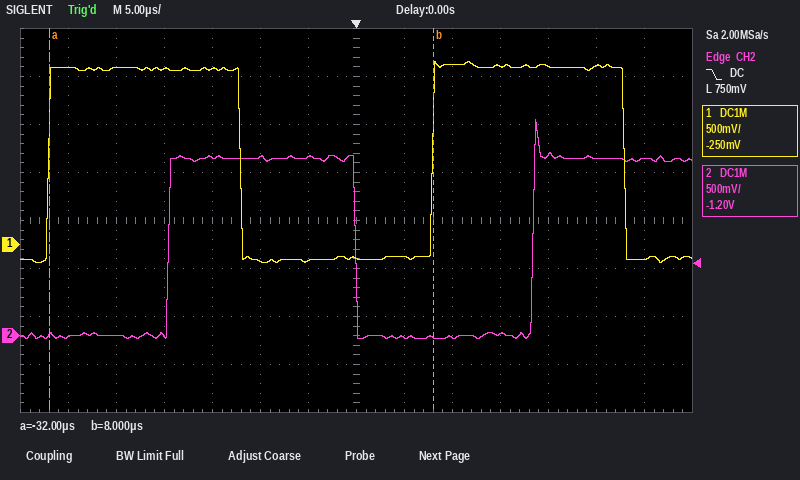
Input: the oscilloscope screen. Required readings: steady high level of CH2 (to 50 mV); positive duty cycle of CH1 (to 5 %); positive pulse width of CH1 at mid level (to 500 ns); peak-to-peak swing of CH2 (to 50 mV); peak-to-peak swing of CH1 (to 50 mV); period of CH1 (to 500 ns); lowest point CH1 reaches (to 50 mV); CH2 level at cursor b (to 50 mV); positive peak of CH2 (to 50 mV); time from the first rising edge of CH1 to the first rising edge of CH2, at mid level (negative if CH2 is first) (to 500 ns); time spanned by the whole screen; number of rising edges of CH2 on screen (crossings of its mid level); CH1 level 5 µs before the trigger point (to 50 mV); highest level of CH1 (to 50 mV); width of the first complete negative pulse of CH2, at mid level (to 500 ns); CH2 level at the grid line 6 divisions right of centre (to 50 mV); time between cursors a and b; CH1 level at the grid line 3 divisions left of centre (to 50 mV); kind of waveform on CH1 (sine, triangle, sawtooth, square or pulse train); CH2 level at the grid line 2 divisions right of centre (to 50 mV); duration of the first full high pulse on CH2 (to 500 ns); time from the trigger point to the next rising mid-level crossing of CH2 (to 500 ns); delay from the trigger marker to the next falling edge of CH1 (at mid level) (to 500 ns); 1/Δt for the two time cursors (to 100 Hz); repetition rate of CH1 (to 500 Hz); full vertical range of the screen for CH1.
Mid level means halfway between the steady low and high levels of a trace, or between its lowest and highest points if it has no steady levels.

1.85 V
50 %
20.0 µs
2.30 V
2.10 V
40.0 µs
-200 mV
0 mV
2.25 V
+12.5 µs
70 µs
2
-150 mV
1.90 V
18.5 µs
1.85 V
40.0 µs
1.85 V
square
0 mV
19.5 µs
18.5 µs
28.0 µs
25.0 kHz
25.0 kHz
4 V
